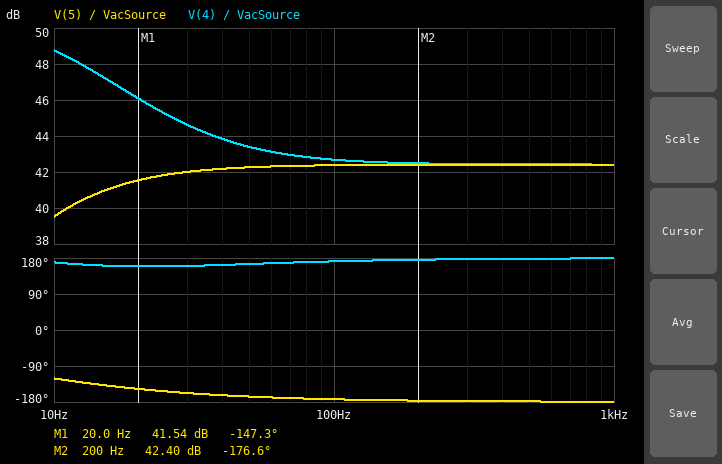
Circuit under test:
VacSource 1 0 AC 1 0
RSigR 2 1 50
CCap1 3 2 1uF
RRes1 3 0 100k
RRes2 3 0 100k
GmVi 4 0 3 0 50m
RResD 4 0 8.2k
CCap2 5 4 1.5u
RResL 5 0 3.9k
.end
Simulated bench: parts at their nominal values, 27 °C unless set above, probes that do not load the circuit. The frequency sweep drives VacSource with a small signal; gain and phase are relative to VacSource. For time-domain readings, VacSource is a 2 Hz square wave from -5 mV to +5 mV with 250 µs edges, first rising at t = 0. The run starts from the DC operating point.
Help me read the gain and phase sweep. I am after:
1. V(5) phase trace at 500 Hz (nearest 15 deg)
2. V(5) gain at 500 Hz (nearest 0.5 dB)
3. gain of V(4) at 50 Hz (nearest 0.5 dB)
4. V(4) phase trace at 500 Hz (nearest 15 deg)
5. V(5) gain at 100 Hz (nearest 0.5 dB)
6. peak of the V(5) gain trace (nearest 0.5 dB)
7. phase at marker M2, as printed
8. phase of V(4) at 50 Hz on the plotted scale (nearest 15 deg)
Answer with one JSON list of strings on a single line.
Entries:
["-180 deg", "42.5 dB", "43.5 dB", "180 deg", "42.5 dB", "42.5 dB", "-176.6 deg", "165 deg"]
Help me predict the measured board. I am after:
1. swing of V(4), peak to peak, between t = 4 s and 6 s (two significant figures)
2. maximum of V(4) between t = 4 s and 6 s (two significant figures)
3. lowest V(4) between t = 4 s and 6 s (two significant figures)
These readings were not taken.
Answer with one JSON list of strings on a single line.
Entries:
["4.7 V", "2.3 V", "-2.3 V"]
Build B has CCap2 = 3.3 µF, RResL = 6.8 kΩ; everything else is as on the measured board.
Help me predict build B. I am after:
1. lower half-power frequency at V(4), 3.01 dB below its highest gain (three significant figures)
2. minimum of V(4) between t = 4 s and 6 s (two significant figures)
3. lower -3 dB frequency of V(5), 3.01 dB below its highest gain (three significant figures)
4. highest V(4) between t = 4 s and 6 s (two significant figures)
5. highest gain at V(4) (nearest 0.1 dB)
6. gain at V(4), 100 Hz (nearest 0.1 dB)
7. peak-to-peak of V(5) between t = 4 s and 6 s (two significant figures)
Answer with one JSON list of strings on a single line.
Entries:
["1.52 Hz", "-1.8 V", "4.97 Hz", "1.8 V", "47.3 dB", "45.4 dB", "3.8 V"]
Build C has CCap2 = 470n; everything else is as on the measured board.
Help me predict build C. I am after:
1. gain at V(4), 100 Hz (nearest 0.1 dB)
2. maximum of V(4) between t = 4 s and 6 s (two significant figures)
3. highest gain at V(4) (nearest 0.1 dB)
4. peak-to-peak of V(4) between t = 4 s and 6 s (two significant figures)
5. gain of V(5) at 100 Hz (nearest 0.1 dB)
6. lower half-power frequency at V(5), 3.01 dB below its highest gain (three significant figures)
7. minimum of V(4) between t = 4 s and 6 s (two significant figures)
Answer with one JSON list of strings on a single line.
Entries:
["44.5 dB", "3.1 V", "51.4 dB", "6.2 V", "42.1 dB", "28.3 Hz", "-3.1 V"]
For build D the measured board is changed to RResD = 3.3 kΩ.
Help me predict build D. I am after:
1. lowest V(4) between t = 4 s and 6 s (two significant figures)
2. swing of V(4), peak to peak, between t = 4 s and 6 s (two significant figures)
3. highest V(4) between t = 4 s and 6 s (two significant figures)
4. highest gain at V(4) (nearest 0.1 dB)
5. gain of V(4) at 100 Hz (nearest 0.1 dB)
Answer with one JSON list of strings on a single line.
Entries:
["-1.1 V", "2.3 V", "1.1 V", "42.9 dB", "39.2 dB"]
